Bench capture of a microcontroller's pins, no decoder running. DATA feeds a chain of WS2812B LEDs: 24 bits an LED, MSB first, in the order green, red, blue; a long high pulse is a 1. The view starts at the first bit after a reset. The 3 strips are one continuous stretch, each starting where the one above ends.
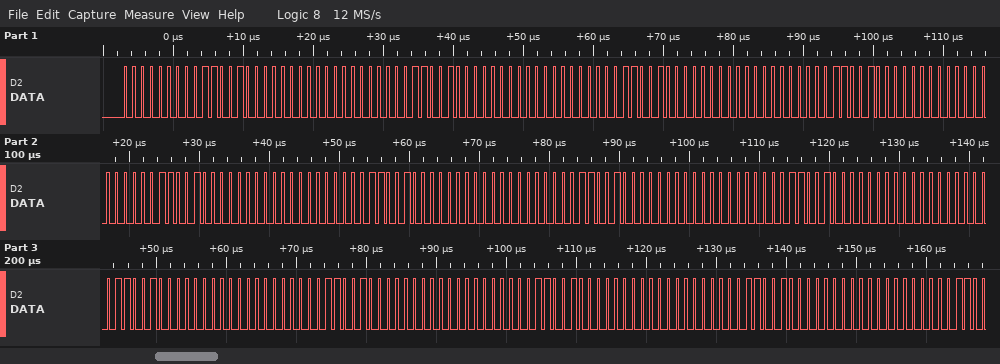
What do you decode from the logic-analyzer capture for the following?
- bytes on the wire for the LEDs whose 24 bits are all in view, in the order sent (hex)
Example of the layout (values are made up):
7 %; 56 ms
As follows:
00 64 00 00 64 00 00 64 00 00 64 00 00 64 00 00 64 00 00 64 00 00 64 00 00 64 00 00 64 00 00 64 00 00 64 00
